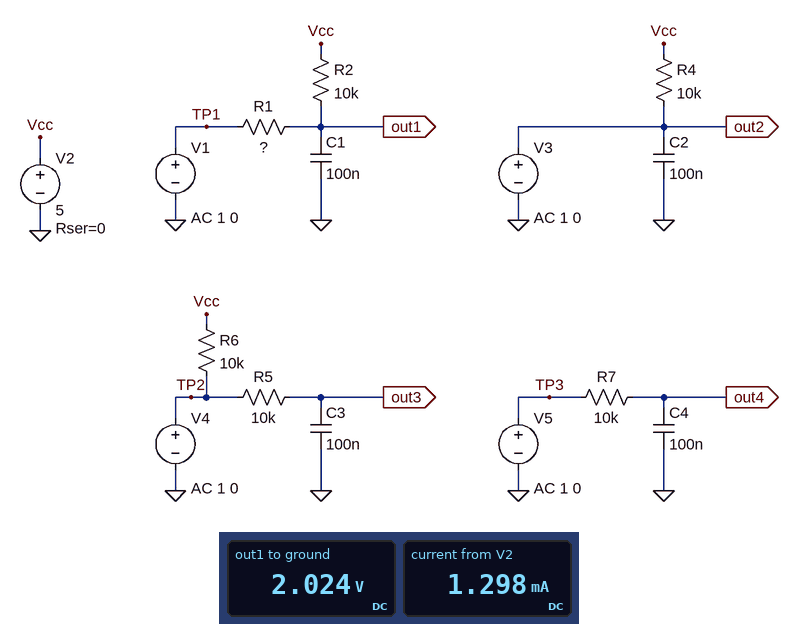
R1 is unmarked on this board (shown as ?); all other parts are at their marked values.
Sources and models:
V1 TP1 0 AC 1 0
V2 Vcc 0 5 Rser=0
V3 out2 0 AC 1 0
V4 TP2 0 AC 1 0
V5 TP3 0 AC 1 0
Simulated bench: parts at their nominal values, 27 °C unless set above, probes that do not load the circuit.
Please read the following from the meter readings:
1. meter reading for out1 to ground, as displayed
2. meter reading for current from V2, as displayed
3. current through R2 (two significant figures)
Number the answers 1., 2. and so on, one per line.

1. 2.024 V
2. 1.298 mA
3. 300 µA
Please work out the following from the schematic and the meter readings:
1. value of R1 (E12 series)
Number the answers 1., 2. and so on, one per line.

1. 6.8 kΩ
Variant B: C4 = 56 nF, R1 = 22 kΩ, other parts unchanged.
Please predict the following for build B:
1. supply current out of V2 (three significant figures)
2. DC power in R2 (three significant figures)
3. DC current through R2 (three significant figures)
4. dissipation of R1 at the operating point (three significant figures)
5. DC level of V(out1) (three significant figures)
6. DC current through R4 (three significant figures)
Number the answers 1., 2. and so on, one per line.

1. 1.16 mA
2. 244 µW
3. 156 µA
4. 537 µW
5. 3.44 V
6. 500 µA
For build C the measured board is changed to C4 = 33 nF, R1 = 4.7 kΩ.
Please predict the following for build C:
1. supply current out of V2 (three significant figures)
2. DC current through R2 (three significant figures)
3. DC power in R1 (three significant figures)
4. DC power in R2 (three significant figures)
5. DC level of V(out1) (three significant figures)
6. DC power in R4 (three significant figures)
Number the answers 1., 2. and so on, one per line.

1. 1.34 mA
2. 340 µA
3. 544 µW
4. 1.16 mW
5. 1.60 V
6. 2.50 mW
